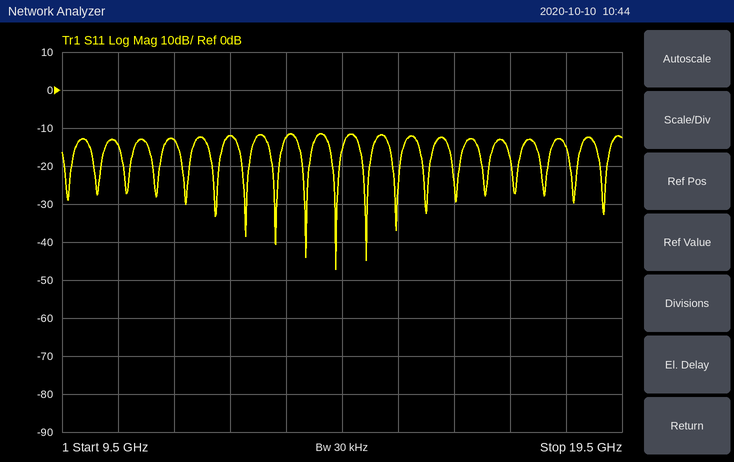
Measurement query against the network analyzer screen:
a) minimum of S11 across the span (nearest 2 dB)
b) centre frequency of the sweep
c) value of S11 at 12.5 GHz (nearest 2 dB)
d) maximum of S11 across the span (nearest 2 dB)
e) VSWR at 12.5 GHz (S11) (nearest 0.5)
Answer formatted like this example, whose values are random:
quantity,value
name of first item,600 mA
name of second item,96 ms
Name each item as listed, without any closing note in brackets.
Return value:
quantity,value
minimum of S11 across the span,-48 dB
centre frequency of the sweep,14.5 GHz
value of S11 at 12.5 GHz,-12 dB
maximum of S11 across the span,-12 dB
VSWR at 12.5 GHz (S11),1.5
